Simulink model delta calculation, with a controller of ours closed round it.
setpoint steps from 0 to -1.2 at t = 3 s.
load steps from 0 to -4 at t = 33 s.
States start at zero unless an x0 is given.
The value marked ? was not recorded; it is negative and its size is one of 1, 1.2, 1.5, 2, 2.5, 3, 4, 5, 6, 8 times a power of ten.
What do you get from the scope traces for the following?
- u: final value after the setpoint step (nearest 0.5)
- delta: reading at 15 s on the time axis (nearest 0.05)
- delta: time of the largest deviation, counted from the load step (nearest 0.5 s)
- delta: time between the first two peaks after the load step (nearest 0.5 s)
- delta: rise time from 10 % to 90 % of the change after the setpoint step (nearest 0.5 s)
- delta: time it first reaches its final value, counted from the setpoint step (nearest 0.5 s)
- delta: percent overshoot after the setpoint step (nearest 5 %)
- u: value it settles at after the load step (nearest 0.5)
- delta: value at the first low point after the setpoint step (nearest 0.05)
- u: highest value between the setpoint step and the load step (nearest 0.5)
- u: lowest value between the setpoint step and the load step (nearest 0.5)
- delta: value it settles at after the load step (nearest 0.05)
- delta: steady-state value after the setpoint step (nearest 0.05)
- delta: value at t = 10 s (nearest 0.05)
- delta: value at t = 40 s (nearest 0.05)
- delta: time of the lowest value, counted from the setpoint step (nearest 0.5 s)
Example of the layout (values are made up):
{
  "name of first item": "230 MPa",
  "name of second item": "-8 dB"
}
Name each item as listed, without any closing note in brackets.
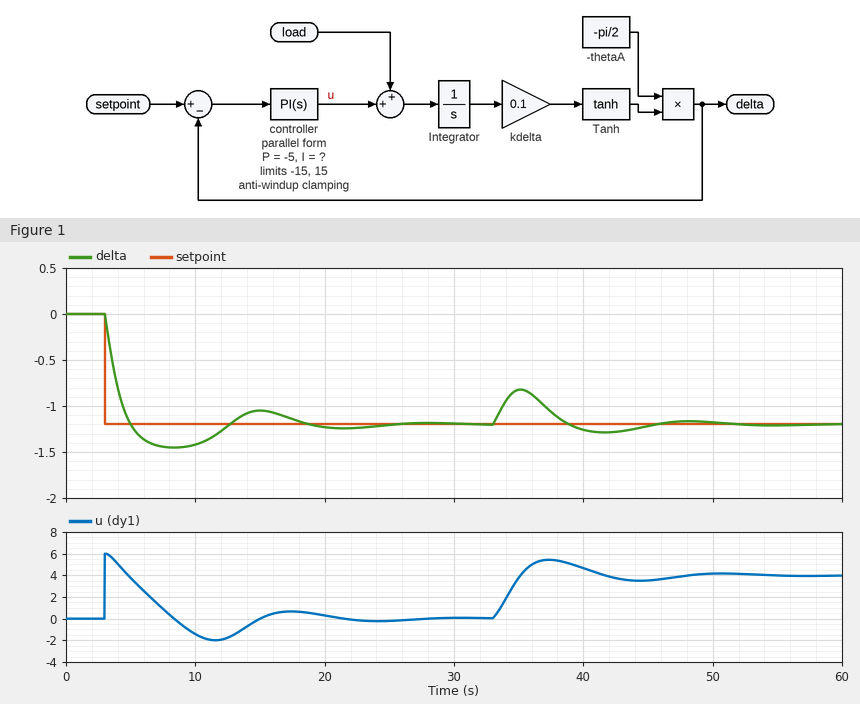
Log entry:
{
  "u: final value after the setpoint step": "0.0",
  "delta: reading at 15 s on the time axis": "-1.05",
  "delta: time of the largest deviation, counted from the load step": "2.0 s",
  "delta: time between the first two peaks after the load step": "13.0 s",
  "delta: rise time from 10 % to 90 % of the change after the setpoint step": "1.5 s",
  "delta: time it first reaches its final value, counted from the setpoint step": "2.0 s",
  "delta: percent overshoot after the setpoint step": "20 %",
  "u: value it settles at after the load step": "4.0",
  "delta: value at the first low point after the setpoint step": "-1.45",
  "u: highest value between the setpoint step and the load step": "6.0",
  "u: lowest value between the setpoint step and the load step": "-2.0",
  "delta: value it settles at after the load step": "-1.20",
  "delta: steady-state value after the setpoint step": "-1.20",
  "delta: value at t = 10 s": "-1.40",
  "delta: value at t = 40 s": "-1.25",
  "delta: time of the lowest value, counted from the setpoint step": "5.5 s"
}
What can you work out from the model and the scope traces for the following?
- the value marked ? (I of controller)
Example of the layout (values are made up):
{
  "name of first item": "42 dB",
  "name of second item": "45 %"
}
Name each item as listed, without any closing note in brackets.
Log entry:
{
  "the value marked ?": "-4"
}
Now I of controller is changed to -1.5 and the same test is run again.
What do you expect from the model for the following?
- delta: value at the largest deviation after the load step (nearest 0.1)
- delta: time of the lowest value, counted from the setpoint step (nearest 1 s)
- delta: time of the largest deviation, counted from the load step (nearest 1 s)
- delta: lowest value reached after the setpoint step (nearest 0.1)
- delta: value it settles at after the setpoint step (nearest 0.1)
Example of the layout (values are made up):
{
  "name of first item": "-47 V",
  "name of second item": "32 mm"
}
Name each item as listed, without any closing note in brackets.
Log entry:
{
  "delta: value at the largest deviation after the load step": "-0.7",
  "delta: time of the lowest value, counted from the setpoint step": "8 s",
  "delta: time of the largest deviation, counted from the load step": "3 s",
  "delta: lowest value reached after the setpoint step": "-1.4",
  "delta: value it settles at after the setpoint step": "-1.2"
}
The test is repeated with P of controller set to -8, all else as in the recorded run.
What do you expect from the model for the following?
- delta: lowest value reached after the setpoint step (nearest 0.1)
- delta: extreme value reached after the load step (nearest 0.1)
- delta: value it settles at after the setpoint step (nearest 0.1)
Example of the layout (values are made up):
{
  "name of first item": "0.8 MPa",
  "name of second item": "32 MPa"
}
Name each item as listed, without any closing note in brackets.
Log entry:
{
  "delta: lowest value reached after the setpoint step": "-1.4",
  "delta: extreme value reached after the load step": "-0.9",
  "delta: value it settles at after the setpoint step": "-1.2"
}
